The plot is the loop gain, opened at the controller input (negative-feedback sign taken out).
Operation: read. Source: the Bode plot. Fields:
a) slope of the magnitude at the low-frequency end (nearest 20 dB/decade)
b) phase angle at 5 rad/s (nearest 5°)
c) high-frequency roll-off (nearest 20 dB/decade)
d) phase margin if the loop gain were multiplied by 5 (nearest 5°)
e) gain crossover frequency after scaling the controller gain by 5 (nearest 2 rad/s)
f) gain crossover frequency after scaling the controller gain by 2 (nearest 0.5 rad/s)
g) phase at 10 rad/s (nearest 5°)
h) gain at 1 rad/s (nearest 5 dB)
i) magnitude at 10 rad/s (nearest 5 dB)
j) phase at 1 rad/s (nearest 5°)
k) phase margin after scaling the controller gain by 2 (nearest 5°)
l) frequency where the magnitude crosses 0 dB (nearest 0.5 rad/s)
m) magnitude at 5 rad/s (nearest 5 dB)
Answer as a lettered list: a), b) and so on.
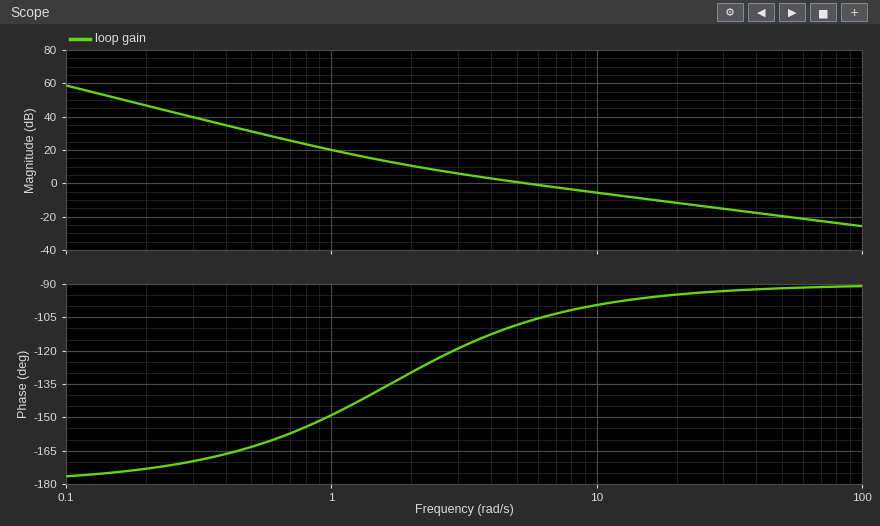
a) -40 dB/decade
b) -110°
c) -20 dB/decade
d) 85°
e) 26 rad/s
f) 10.5 rad/s
g) -100°
h) 20 dB
i) -5 dB
j) -150°
k) 80°
l) 5.5 rad/s
m) 0 dB
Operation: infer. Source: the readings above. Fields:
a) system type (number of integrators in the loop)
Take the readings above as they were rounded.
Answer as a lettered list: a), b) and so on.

a) 2
